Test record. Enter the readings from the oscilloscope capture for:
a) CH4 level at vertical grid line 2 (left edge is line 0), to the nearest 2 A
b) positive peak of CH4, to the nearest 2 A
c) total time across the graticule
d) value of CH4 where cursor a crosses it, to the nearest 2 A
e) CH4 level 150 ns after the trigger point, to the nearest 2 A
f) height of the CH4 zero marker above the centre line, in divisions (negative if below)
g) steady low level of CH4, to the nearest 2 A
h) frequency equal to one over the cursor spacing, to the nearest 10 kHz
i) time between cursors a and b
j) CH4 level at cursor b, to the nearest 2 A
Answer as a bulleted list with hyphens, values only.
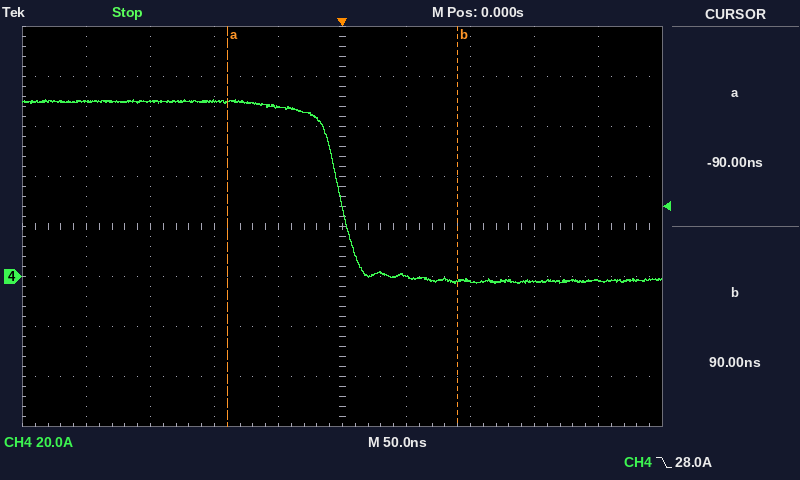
- 70 A
- 70 A
- 500 ns
- 70 A
- -2 A
- -1.0 div
- -2 A
- 5.56 MHz
- 180 ns
- -2 A
